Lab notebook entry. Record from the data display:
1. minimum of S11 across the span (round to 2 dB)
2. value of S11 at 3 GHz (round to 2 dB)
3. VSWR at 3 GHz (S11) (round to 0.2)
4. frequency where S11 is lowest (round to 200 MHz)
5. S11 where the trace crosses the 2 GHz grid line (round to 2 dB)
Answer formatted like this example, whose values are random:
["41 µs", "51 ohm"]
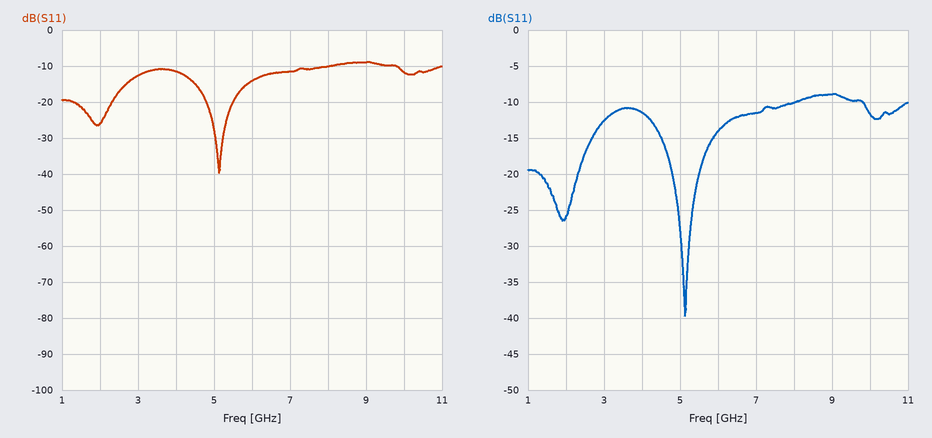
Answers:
["-40 dB", "-12 dB", "1.6", "5.2 GHz", "-26 dB"]
